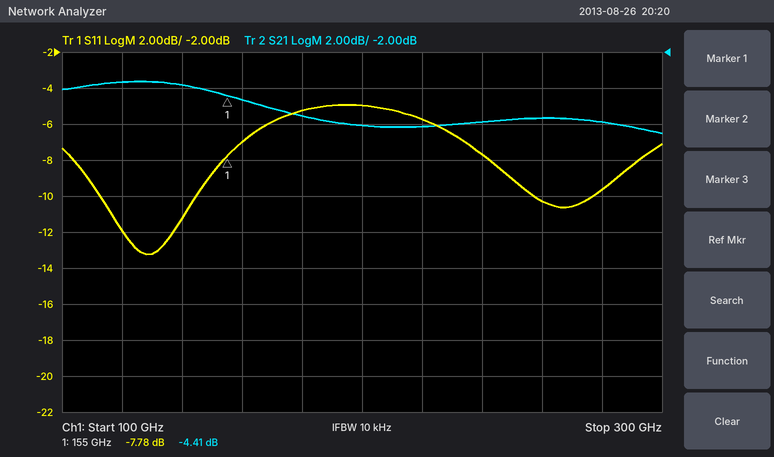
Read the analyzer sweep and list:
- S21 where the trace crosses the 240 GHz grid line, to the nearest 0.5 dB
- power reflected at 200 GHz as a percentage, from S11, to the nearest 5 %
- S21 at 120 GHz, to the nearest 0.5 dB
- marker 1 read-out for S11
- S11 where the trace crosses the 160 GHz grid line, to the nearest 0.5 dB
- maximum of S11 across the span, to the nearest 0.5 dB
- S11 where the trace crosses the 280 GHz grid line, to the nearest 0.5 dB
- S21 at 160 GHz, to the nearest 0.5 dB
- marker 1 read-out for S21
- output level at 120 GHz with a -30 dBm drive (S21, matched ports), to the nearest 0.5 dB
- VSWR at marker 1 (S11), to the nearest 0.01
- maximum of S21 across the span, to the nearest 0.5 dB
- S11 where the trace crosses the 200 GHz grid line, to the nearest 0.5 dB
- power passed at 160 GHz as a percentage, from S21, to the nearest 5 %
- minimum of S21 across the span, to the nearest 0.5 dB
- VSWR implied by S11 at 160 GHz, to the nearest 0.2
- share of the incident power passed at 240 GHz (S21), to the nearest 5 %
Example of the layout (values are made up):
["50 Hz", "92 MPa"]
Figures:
["-6.0 dB", "30 %", "-3.5 dB", "-7.78 dB", "-7.0 dB", "-5.0 dB", "-9.5 dB", "-4.5 dB", "-4.41 dB", "-33.5 dBm", "2.38", "-3.5 dB", "-5.0 dB", "35 %", "-6.5 dB", "2.6", "25 %"]
